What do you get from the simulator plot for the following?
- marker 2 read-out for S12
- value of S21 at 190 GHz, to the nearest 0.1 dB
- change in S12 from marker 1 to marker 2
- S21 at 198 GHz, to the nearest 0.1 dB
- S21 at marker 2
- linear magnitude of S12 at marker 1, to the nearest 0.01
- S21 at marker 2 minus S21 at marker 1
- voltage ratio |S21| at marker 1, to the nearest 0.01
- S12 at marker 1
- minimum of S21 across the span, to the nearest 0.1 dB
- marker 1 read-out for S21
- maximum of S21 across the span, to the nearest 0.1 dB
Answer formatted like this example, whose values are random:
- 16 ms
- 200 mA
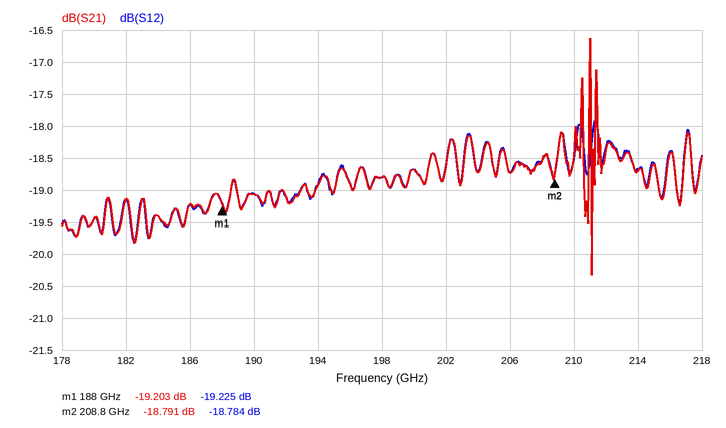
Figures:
- -18.784 dB
- -19.1 dB
- 0.441 dB
- -18.8 dB
- -18.791 dB
- 0.11
- 0.412 dB
- 0.11
- -19.225 dB
- -20.3 dB
- -19.203 dB
- -16.6 dB
